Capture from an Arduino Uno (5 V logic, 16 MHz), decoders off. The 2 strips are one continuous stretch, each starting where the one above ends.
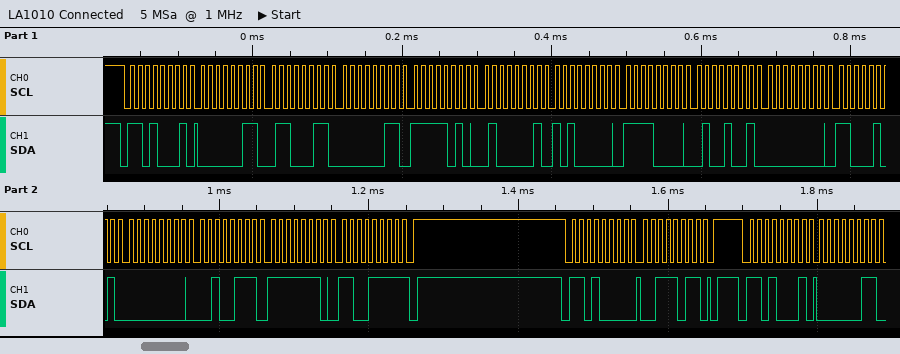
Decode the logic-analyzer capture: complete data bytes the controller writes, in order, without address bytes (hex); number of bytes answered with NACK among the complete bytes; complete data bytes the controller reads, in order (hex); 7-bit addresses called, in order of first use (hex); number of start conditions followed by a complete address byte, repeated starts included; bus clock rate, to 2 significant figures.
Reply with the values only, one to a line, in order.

3B
1
03 63 03 FA 41 A0 F0 49 00 C5 00 27 FE CF 03
0x68
3
100 kHz
